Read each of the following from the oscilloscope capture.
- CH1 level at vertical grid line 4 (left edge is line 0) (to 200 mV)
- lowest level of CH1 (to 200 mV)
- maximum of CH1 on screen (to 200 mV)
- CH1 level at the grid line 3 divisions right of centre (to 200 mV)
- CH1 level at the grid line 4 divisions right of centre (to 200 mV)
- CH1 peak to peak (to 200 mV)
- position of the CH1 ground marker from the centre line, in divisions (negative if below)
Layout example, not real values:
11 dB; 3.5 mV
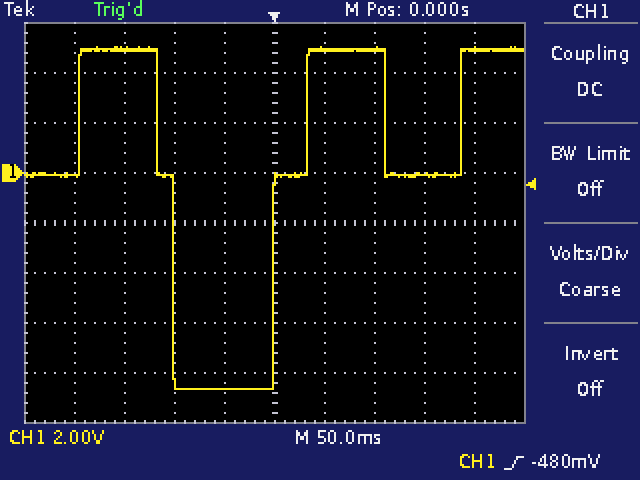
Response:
-8.6 V; -8.6 V; 5.0 V; 0.0 V; 5.0 V; 13.6 V; +1.0 div
